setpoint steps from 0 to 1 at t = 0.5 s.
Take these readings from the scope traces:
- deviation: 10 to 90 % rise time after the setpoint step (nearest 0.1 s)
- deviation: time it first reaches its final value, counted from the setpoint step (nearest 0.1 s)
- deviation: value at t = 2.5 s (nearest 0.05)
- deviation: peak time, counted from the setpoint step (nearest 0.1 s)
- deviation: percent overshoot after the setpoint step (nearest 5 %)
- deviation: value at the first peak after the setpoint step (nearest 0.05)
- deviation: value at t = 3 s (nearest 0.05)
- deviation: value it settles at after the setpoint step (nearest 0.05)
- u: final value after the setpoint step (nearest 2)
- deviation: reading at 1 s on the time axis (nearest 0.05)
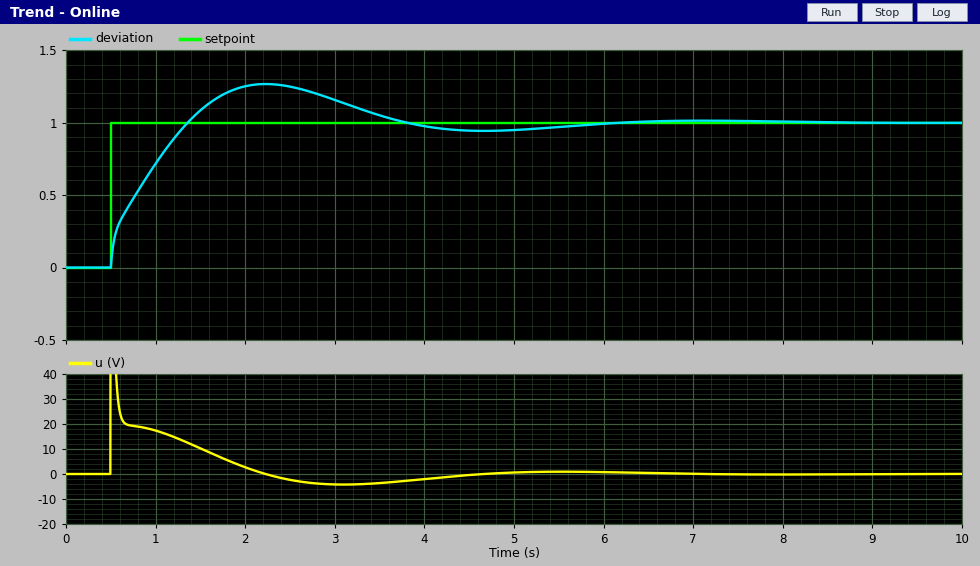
0.7 s
0.9 s
1.25
1.7 s
25 %
1.25
1.15
1.00
0
0.70
